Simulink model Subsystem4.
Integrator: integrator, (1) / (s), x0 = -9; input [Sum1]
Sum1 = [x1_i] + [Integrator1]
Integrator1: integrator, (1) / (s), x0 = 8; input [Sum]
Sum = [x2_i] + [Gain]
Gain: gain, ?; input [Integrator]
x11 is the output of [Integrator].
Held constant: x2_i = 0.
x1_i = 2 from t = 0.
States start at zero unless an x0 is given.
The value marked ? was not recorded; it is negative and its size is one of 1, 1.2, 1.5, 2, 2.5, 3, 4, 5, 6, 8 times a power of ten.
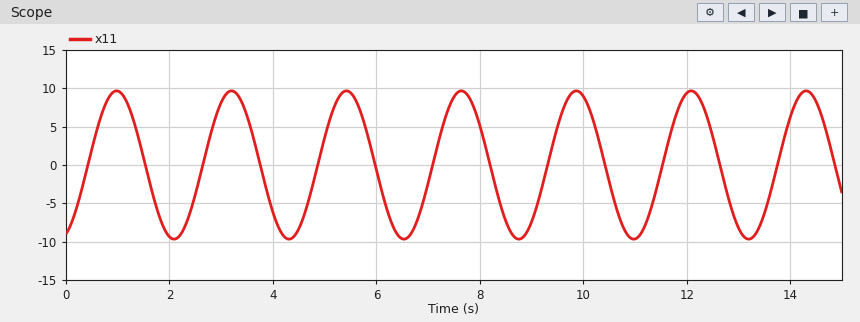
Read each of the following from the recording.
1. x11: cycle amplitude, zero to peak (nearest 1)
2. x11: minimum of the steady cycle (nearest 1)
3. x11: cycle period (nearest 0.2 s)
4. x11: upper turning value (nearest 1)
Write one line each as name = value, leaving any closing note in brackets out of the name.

x11: cycle amplitude, zero to peak = 10
x11: minimum of the steady cycle = -10
x11: cycle period = 2.2 s
x11: upper turning value = 10
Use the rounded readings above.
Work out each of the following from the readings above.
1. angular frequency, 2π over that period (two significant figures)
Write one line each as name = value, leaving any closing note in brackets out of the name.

angular frequency, 2π over that period = 2.9 rad/s
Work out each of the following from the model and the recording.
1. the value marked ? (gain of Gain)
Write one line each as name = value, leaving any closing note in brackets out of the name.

the value marked ? = -8
